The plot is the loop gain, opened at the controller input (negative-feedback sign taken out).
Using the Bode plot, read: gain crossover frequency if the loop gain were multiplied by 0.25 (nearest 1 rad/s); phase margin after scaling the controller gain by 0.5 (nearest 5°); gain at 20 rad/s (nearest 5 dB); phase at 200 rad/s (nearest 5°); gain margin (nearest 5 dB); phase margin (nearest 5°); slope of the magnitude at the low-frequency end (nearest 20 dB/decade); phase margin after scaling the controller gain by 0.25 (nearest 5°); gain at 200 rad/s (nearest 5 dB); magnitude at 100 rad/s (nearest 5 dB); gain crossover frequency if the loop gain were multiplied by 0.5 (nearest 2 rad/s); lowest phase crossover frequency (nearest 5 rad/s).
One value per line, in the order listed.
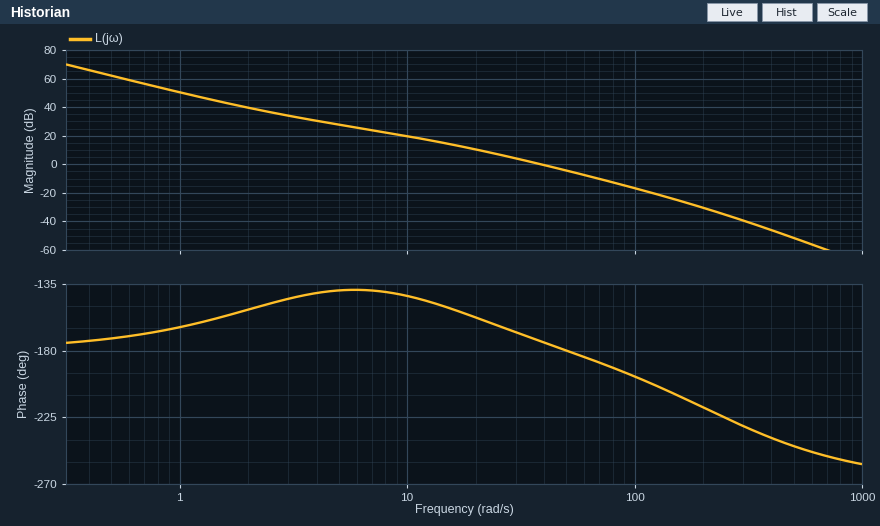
18 rad/s
15°
10 dB
-220°
5 dB
5°
-40 dB/decade
25°
-30 dB
-15 dB
26 rad/s
50 rad/s
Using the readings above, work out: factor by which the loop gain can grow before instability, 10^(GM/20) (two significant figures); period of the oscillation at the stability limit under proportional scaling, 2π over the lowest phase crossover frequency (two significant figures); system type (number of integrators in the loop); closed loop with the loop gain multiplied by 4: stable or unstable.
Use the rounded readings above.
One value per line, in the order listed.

1.8
0.13 s
2
unstable
